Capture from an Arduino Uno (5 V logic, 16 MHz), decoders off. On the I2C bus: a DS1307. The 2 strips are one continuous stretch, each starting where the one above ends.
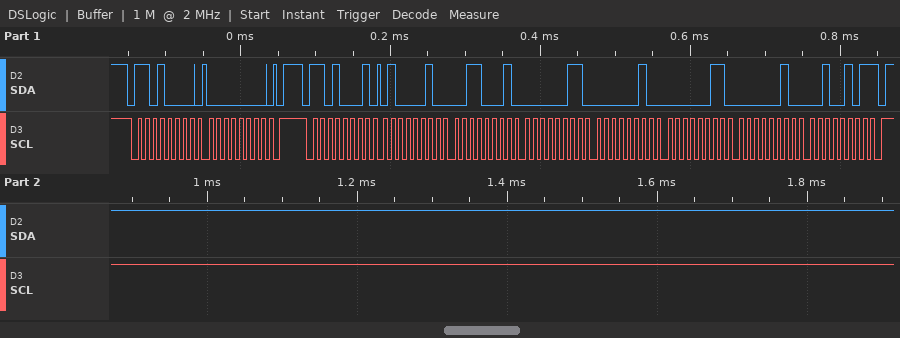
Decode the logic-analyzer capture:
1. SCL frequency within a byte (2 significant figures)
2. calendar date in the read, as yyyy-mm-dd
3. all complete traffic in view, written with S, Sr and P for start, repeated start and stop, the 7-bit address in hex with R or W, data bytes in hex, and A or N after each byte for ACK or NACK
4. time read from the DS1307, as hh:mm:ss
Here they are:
100 kHz
2025-02-03
S 68W A 00 A P S 68R A 42 A 31 A 03 A 02 A 03 A 02 A 25 N P
03:31:42
